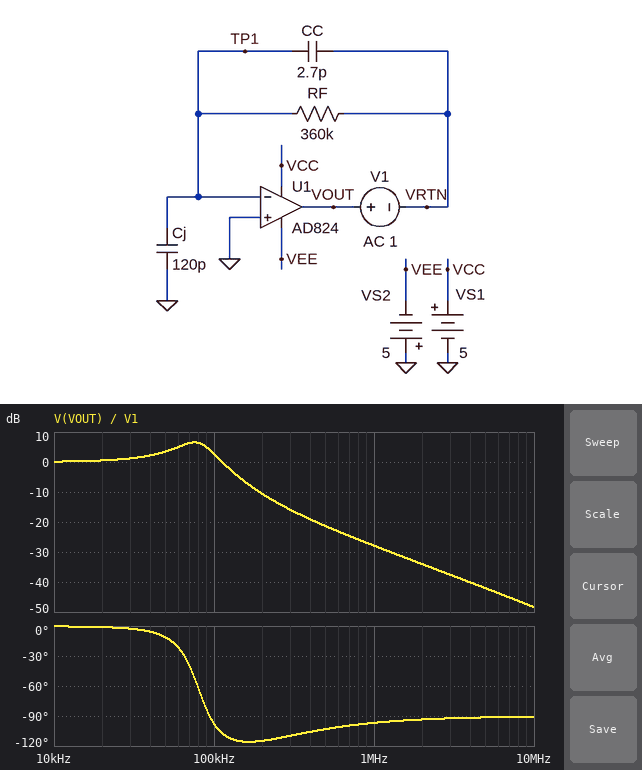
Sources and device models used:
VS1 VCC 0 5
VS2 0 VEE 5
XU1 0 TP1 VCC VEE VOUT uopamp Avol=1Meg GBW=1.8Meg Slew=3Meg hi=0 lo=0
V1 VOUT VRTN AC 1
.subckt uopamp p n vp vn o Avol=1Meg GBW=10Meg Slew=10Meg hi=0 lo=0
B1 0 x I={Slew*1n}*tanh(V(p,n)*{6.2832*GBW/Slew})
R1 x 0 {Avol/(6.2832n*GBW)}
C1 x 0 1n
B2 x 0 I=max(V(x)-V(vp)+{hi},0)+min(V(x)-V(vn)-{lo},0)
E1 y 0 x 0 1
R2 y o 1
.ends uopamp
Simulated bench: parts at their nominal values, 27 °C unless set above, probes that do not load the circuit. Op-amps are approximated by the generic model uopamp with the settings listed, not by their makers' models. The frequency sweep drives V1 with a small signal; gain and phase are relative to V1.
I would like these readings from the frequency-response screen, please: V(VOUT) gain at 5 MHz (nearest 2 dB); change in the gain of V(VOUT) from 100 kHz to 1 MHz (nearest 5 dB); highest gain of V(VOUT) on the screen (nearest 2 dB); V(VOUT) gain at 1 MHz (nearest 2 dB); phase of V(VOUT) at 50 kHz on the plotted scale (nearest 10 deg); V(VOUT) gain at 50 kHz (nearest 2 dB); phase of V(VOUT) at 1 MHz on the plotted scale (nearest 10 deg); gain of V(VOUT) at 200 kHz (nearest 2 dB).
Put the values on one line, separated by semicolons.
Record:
-42 dB; -30 dB; 6 dB; -28 dB; -10 deg; 4 dB; -100 deg; -10 dB
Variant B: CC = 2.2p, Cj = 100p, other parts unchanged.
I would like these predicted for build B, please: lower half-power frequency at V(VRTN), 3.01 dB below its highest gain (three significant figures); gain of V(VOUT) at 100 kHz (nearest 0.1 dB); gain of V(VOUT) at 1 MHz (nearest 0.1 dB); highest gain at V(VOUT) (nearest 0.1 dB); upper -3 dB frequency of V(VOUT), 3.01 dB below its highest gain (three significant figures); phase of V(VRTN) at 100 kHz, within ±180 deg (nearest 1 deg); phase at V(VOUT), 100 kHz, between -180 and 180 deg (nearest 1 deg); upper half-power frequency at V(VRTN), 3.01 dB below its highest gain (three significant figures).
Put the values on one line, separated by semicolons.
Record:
75.8 kHz; 5.1 dB; -28.0 dB; 7.2 dB; 104 kHz; -120 deg; -91 deg; 138 kHz
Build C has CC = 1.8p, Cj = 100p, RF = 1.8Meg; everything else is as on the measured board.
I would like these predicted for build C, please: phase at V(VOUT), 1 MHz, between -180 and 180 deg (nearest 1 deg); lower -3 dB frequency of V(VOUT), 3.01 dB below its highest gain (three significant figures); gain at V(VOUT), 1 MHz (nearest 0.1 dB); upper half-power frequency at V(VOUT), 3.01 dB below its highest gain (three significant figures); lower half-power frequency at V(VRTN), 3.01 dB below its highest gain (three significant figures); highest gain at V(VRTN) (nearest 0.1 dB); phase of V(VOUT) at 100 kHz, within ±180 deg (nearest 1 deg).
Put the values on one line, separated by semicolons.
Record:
-91 deg; 14.5 kHz; -29.9 dB; 51.3 kHz; 33.3 kHz; 2.5 dB; -95 deg
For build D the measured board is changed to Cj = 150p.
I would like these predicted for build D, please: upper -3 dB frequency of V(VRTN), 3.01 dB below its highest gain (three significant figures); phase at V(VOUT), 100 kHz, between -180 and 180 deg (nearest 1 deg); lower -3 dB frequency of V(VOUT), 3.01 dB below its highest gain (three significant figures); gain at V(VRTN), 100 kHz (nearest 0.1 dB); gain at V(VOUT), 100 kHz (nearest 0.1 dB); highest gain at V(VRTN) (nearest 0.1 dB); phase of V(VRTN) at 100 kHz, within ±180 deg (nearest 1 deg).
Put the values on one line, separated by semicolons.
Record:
112 kHz; -113 deg; 48.6 kHz; 4.6 dB; 0.3 dB; 6.6 dB; -146 deg
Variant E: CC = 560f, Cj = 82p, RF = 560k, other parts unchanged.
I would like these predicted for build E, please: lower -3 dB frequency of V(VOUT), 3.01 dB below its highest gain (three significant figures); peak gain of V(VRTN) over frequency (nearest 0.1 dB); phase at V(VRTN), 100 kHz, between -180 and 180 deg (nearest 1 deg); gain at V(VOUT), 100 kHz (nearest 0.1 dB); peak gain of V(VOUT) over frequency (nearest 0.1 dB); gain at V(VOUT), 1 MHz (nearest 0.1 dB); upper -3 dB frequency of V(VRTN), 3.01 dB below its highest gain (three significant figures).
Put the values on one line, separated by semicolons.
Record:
69.7 kHz; 14.1 dB; -160 deg; 3.7 dB; 14.2 dB; -37.2 dB; 89.0 kHz
